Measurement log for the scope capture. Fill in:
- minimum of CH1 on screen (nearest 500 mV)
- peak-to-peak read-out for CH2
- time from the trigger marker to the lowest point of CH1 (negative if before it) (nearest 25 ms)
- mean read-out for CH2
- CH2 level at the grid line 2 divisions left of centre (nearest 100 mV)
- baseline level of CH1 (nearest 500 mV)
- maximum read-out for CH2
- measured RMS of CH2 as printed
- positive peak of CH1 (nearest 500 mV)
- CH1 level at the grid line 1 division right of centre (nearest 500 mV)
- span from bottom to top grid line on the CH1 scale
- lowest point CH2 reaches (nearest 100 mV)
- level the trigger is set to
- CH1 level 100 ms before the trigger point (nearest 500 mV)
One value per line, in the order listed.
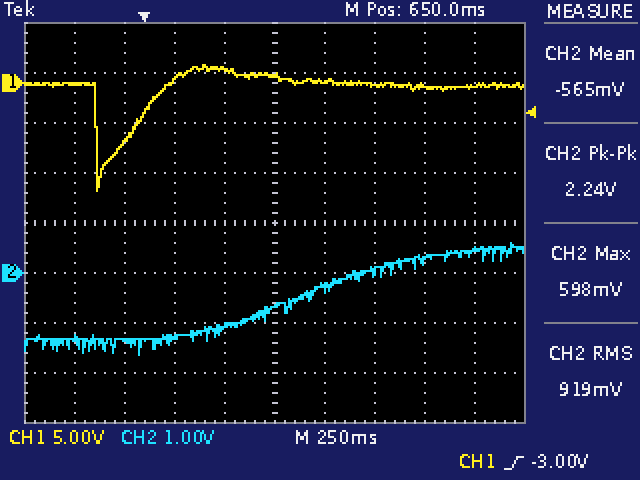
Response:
-11.0 V
2.24 V
-225 ms
-565 mV
-1.3 V
0.0 V
598 mV
919 mV
2.0 V
0.0 V
40 V
-1.6 V
-3.00 V
-6.0 V
